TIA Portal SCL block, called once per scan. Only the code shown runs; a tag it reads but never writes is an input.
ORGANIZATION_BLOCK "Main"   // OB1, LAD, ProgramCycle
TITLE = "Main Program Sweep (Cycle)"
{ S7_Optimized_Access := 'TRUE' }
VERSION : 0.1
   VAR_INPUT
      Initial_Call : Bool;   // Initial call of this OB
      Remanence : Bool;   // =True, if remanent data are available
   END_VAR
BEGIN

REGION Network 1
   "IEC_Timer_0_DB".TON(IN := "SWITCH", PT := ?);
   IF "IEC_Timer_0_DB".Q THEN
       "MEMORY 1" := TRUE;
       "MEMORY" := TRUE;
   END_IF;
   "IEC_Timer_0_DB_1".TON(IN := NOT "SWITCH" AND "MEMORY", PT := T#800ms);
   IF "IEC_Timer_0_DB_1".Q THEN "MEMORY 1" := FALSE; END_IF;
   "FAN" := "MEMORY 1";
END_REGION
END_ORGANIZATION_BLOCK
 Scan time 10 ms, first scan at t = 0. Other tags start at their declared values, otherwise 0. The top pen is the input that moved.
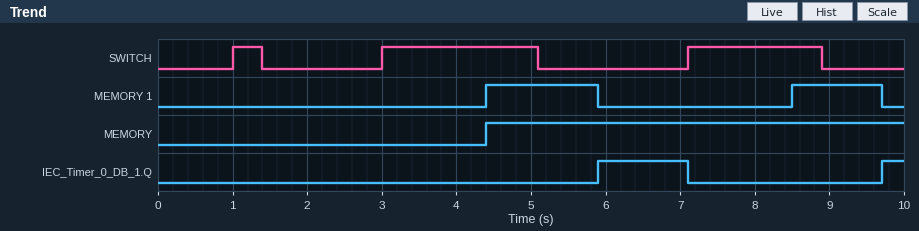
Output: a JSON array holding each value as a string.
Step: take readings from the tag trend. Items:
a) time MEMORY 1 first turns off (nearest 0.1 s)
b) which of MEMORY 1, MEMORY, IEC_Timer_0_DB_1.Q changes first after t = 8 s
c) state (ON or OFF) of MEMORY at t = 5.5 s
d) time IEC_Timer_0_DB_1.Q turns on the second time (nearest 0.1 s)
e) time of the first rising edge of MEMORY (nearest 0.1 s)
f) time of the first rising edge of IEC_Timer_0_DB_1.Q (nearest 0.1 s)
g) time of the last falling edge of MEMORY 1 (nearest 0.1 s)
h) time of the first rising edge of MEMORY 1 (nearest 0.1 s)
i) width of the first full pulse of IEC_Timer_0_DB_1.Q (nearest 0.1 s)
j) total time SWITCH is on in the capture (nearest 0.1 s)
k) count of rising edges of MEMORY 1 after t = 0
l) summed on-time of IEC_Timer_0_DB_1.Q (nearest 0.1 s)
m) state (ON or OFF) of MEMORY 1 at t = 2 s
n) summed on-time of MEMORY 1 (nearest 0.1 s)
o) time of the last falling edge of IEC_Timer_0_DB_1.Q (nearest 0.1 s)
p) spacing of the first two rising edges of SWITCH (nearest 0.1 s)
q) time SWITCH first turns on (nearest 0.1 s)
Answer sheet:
["5.9 s", "MEMORY 1", "ON", "9.7 s", "4.4 s", "5.9 s", "9.7 s", "4.4 s", "1.2 s", "4.3 s", "2", "1.5 s", "OFF", "2.7 s", "7.1 s", "2.0 s", "1.0 s"]
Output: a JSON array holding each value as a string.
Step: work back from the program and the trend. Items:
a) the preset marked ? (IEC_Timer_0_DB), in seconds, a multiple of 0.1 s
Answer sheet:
["1.4 s"]
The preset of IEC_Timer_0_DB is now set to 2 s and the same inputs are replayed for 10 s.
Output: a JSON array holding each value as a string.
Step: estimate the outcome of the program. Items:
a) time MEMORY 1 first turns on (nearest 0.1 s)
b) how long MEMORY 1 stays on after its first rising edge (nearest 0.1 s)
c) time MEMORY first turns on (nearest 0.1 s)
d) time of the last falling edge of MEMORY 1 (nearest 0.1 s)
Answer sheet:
["5.0 s", "0.9 s", "5.0 s", "5.9 s"]
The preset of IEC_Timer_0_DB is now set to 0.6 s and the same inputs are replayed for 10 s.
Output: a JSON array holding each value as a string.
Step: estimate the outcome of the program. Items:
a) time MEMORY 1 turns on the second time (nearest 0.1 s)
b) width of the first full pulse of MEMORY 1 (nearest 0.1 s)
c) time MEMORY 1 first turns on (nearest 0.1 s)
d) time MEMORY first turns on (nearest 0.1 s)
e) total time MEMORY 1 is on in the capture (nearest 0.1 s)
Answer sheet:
["7.7 s", "2.3 s", "3.6 s", "3.6 s", "4.3 s"]
